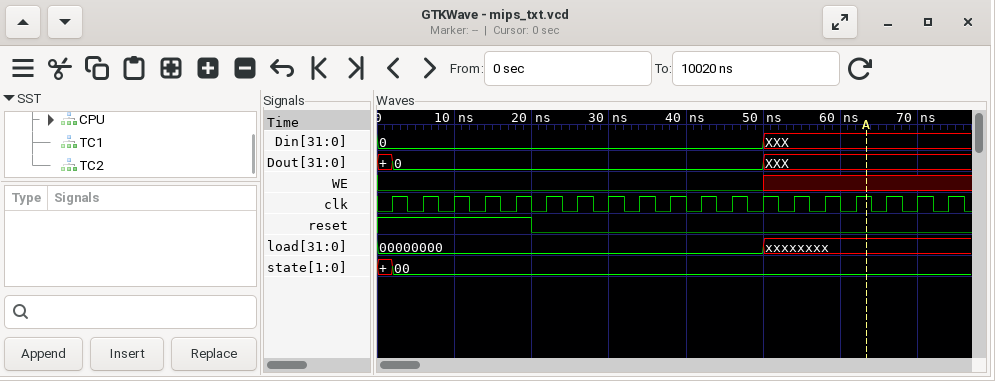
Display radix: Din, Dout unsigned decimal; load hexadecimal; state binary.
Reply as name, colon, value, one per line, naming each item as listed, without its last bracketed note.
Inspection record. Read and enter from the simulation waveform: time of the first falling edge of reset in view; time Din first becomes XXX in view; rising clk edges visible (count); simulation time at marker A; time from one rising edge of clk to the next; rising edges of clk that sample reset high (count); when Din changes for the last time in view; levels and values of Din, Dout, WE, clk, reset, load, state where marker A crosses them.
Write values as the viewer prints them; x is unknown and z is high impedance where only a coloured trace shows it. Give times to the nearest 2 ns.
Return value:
time of the first falling edge of reset in view: 20 ns
time Din first becomes XXX in view: 50 ns
rising clk edges visible: 19
simulation time at marker A: 64 ns
time from one rising edge of clk to the next: 4 ns
rising edges of clk that sample reset high: 5
when Din changes for the last time in view: 50 ns
levels and values of Din, Dout, WE, clk, reset, load, state where marker A crosses them: Din=XXX, Dout=XXX, WE=x, clk=1, reset=0, load=xxxxxxxx, state=00
